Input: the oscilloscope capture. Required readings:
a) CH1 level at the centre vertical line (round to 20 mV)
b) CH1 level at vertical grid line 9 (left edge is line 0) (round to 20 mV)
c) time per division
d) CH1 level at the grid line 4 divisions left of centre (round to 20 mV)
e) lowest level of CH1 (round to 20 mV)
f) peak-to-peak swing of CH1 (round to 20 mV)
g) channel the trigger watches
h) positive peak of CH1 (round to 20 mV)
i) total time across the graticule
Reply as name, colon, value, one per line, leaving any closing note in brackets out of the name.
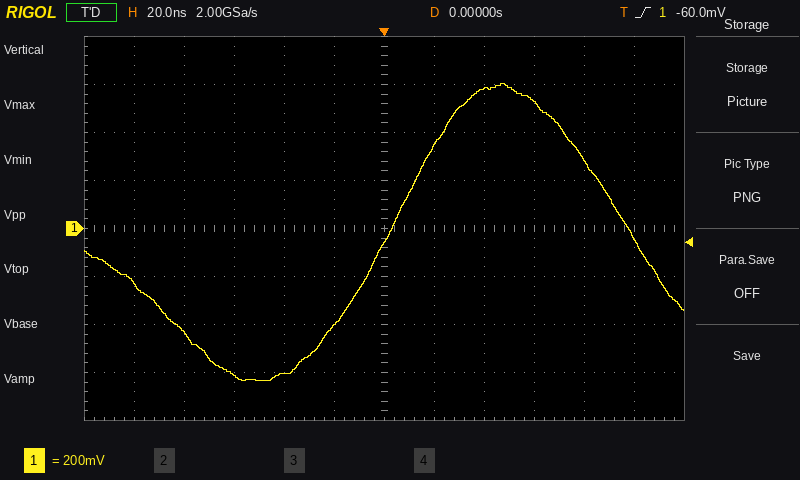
CH1 level at the centre vertical line: -60 mV
CH1 level at vertical grid line 9 (left edge is line 0): 520 mV
time per division: 20 ns
CH1 level at the grid line 4 divisions left of centre: -440 mV
lowest level of CH1: -640 mV
peak-to-peak swing of CH1: 1.24 V
channel the trigger watches: CH1
positive peak of CH1: 600 mV
total time across the graticule: 240 ns
